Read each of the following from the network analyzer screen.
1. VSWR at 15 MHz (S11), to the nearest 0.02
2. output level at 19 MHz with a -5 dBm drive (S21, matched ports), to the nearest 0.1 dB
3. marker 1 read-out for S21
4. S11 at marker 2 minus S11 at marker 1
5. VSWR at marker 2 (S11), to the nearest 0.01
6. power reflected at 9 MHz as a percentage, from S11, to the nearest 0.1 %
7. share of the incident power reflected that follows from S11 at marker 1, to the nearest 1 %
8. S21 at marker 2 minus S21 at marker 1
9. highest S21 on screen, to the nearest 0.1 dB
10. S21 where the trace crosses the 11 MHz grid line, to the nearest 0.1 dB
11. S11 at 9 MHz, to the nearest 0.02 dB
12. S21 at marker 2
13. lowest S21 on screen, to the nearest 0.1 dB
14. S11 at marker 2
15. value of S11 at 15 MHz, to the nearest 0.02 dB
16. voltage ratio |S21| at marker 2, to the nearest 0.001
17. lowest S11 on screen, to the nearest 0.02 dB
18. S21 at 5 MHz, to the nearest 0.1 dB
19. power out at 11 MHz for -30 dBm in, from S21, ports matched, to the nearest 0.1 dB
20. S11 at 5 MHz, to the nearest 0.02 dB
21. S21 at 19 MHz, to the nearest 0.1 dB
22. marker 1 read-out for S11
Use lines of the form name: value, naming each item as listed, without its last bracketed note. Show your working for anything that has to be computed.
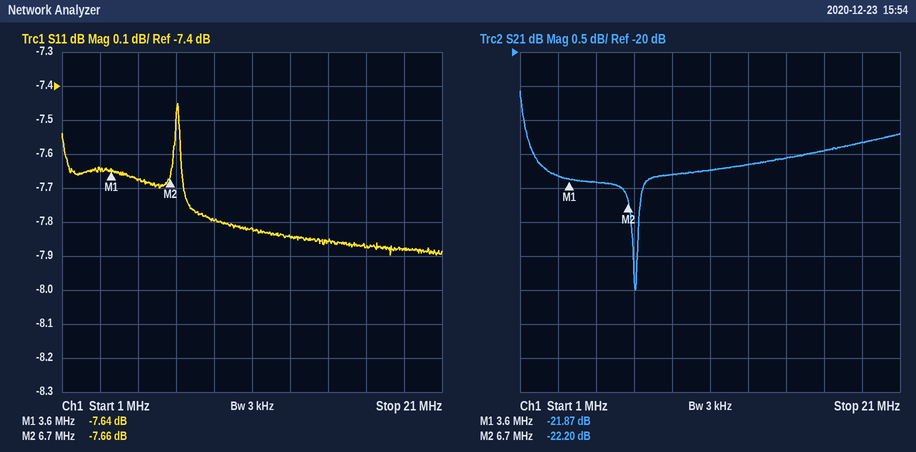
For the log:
VSWR at 15 MHz (S11), to the nearest 0.02: |Γ| = 10^(-7.86/20) = 0.4046; VSWR = (1 + 0.4046)/(1 − 0.4046) ≈ 2.36
output level at 19 MHz with a -5 dBm drive (S21, matched ports), to the nearest 0.1 dB: -5 dBm + (-21.3 dB) = -26.3 dBm
marker 1 read-out for S21: -21.87 dB
S11 at marker 2 minus S11 at marker 1: -7.66 − (-7.64) = -0.02 dB
VSWR at marker 2 (S11), to the nearest 0.01: (1 + 0.4140)/(1 − 0.4140) ≈ 2.41
power reflected at 9 MHz as a percentage, from S11, to the nearest 0.1 %: 10^(-7.8/10) ≈ 16.6 %
share of the incident power reflected that follows from S11 at marker 1, to the nearest 1 %: 10^(-7.64/10) ≈ 17 %
S21 at marker 2 minus S21 at marker 1: -22.2 − (-21.87) = -0.33 dB
highest S21 on screen, to the nearest 0.1 dB: -20.6 dB
S21 where the trace crosses the 11 MHz grid line, to the nearest 0.1 dB: -21.7 dB
S11 at 9 MHz, to the nearest 0.02 dB: -7.80 dB
S21 at marker 2: -22.20 dB
lowest S21 on screen, to the nearest 0.1 dB: -23.5 dB
S11 at marker 2: -7.66 dB
value of S11 at 15 MHz, to the nearest 0.02 dB: -7.86 dB
voltage ratio |S21| at marker 2, to the nearest 0.001: 10^(-22.2/20) ≈ 0.078
lowest S11 on screen, to the nearest 0.02 dB: -7.90 dB
S21 at 5 MHz, to the nearest 0.1 dB: -21.9 dB
power out at 11 MHz for -30 dBm in, from S21, ports matched, to the nearest 0.1 dB: -30 dBm + (-21.7 dB) = -51.7 dBm
S11 at 5 MHz, to the nearest 0.02 dB: -7.68 dB
S21 at 19 MHz, to the nearest 0.1 dB: -21.3 dB
marker 1 read-out for S11: -7.64 dB
